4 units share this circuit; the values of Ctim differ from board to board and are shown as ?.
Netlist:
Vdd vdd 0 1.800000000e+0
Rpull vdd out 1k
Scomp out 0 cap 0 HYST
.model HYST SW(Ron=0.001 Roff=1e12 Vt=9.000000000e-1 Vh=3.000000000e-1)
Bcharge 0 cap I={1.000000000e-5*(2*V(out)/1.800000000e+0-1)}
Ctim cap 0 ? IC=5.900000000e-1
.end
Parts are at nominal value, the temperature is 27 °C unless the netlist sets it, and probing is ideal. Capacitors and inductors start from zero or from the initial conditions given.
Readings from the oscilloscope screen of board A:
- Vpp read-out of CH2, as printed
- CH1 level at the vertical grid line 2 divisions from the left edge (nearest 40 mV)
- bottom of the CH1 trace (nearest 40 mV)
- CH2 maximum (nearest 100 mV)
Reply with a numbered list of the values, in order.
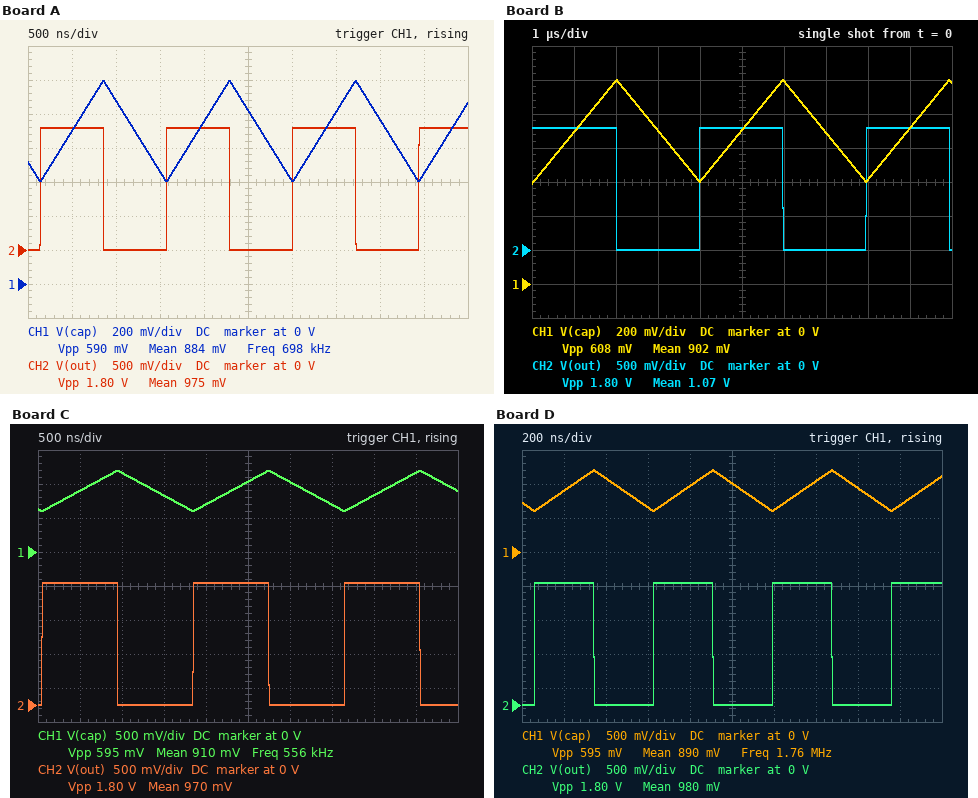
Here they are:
1. 1.80 V
2. 1.08 V
3. 600 mV
4. 1.8 V
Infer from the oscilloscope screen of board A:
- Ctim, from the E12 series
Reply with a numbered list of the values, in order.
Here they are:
1. 12 pF
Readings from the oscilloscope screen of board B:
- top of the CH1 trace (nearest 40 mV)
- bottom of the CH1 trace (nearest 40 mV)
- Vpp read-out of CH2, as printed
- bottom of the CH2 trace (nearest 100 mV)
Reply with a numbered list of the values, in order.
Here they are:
1. 1.20 V
2. 600 mV
3. 1.80 V
4. 0 V
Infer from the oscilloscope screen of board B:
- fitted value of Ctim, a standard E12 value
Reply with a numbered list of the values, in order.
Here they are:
1. 33 pF
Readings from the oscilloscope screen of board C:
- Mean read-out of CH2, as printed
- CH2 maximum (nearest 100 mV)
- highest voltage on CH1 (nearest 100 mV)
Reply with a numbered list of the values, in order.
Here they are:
1. 970 mV
2. 1.8 V
3. 1.2 V
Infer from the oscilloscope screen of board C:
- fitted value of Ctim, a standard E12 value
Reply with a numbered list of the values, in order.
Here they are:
1. 15 pF
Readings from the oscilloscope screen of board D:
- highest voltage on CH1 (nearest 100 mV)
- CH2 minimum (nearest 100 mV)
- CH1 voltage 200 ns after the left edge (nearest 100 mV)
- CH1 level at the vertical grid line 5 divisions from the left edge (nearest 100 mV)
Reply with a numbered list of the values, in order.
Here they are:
1. 1.2 V
2. 0 V
3. 900 mV
4. 1.0 V
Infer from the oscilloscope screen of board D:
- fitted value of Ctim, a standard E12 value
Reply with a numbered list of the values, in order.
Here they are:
1. 4.7 pF
